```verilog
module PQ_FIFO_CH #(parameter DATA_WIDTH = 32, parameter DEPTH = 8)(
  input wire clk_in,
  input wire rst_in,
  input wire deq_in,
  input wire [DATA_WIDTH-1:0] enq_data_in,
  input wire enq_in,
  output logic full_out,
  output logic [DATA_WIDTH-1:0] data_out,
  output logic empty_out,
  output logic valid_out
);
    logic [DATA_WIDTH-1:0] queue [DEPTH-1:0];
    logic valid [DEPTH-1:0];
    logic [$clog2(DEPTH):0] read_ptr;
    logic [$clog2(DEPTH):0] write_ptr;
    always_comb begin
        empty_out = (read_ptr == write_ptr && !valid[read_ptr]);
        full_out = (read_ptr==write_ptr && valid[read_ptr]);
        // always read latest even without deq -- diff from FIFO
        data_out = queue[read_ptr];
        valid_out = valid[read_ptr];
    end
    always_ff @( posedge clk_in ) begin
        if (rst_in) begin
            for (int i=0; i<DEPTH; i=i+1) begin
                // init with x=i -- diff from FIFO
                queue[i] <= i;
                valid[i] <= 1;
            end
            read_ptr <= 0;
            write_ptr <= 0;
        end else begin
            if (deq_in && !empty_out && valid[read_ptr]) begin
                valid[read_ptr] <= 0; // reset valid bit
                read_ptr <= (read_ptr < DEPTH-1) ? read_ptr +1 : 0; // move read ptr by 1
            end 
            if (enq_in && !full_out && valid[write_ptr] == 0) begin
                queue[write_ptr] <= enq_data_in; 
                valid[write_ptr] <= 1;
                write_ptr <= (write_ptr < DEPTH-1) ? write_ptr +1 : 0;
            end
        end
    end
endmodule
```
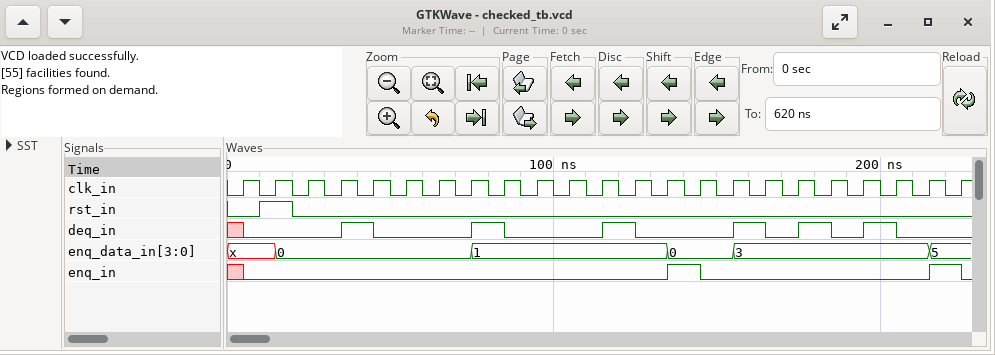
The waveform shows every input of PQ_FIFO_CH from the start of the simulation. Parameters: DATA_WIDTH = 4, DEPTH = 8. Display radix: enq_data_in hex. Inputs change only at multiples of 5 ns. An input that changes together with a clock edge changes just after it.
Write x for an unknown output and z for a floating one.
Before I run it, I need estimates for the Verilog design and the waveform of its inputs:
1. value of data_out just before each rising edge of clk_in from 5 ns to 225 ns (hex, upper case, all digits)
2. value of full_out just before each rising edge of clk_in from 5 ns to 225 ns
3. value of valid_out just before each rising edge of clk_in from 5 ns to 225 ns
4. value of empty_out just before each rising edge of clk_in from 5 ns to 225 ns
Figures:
x, x, 0, 0, 0, 1, 1, 1, 1, 2, 2, 2, 2, 3, 3, 3, 3, 4, 4, 5, 5, 6, 6
x x 1 1 1 0 0 0 0 0 0 0 0 0 0 0 0 0 0 0 0 0 0
x x 1 1 1 1 1 1 1 1 1 1 1 1 1 1 1 1 1 1 1 1 1
x x 0 0 0 0 0 0 0 0 0 0 0 0 0 0 0 0 0 0 0 0 0
